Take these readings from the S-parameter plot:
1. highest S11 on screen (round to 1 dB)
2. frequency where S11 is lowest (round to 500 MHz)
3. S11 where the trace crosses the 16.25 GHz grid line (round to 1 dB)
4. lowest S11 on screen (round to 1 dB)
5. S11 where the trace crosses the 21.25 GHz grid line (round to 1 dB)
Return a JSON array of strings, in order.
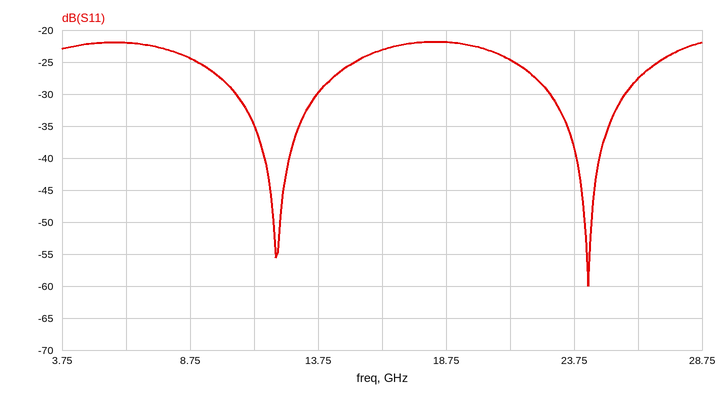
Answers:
["-22 dB", "24.5 GHz", "-23 dB", "-60 dB", "-25 dB"]
